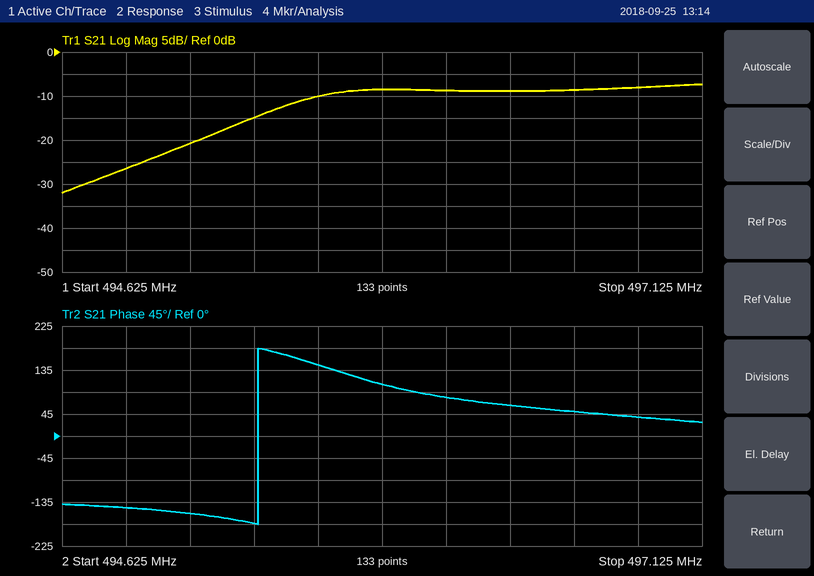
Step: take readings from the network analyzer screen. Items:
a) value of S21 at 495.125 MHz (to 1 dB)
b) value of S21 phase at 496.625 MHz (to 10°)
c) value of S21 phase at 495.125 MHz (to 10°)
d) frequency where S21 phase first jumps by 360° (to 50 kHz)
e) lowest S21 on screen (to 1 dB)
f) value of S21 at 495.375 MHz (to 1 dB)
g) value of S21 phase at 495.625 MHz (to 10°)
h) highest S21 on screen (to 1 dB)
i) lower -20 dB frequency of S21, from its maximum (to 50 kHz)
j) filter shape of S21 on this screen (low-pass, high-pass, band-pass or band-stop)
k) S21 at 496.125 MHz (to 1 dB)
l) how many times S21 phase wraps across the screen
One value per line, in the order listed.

-21 dB
50°
-160°
495.40 MHz
-32 dB
-15 dB
150°
-7 dB
494.85 MHz
high-pass
-9 dB
1
